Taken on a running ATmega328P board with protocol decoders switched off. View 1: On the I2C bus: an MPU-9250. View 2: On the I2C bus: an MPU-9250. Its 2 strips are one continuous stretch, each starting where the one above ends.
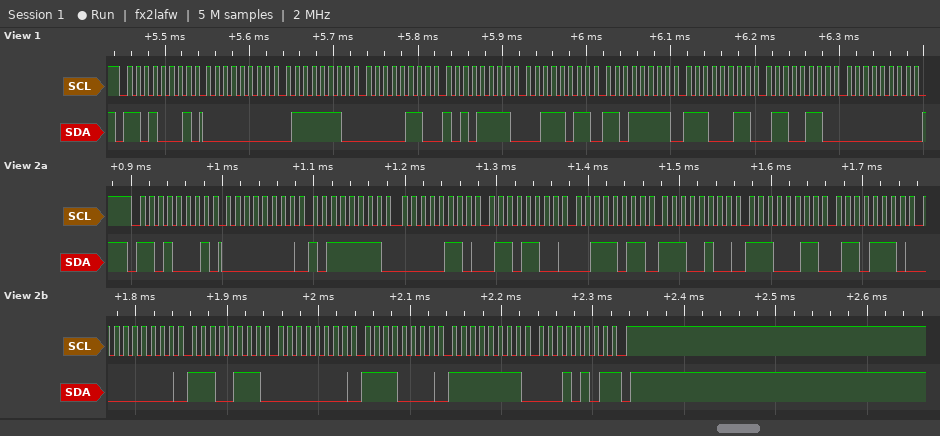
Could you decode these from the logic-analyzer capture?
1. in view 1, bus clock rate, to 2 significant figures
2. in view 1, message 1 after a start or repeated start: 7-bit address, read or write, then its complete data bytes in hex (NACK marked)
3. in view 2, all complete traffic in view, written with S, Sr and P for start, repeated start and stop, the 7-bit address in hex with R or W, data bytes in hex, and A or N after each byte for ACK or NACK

100 kHz
0x68 read: 00 7E 06 AF 3B DF E3 66 00
S 68R A 00 A BF A 06 A 6C A 3B A E4 A E3 A 6E A 00 A E7 A 00 A F0 A FF A 15 N P
